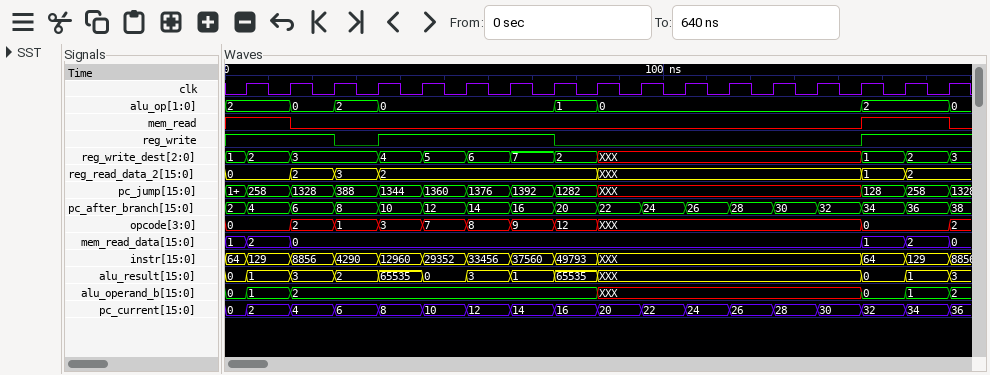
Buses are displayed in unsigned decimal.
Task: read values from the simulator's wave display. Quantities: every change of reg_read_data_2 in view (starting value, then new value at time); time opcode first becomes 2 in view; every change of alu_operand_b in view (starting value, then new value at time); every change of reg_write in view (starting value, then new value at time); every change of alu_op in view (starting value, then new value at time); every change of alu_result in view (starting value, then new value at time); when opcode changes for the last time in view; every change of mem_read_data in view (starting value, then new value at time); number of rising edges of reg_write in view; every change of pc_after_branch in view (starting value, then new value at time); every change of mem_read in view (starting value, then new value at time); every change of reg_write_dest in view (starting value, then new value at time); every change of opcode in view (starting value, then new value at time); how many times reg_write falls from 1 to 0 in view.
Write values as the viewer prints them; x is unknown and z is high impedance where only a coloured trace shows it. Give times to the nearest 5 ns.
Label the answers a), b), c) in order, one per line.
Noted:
a) 0, 2 at 15 ns, 3 at 25 ns, 2 at 35 ns, XXX at 85 ns, 1 at 145 ns, 2 at 155 ns
b) 15 ns
c) 0, 1 at 5 ns, 2 at 15 ns, XXX at 85 ns, 0 at 145 ns, 1 at 155 ns, 2 at 165 ns
d) 1, 0 at 25 ns, 1 at 35 ns, 0 at 75 ns, 1 at 145 ns
e) 2, 0 at 15 ns, 2 at 25 ns, 0 at 35 ns, 1 at 75 ns, 0 at 85 ns, 2 at 145 ns, 0 at 165 ns
f) 0, 1 at 5 ns, 3 at 15 ns, 2 at 25 ns, 65535 at 35 ns, 0 at 45 ns, 3 at 55 ns, 1 at 65 ns, 65535 at 75 ns, XXX at 85 ns, 0 at 145 ns, 1 at 155 ns, 3 at 165 ns
g) 165 ns
h) 1, 2 at 5 ns, 0 at 15 ns, 1 at 145 ns, 2 at 155 ns, 0 at 165 ns
i) 2
j) 2, 4 at 5 ns, 6 at 15 ns, 8 at 25 ns, 10 at 35 ns, 12 at 45 ns, 14 at 55 ns, 16 at 65 ns, 20 at 75 ns, 22 at 85 ns, 24 at 95 ns, 26 at 105 ns, 28 at 115 ns, 30 at 125 ns, 32 at 135 ns, 34 at 145 ns, 36 at 155 ns, 38 at 165 ns
k) 1, 0 at 15 ns, 1 at 145 ns, 0 at 165 ns
l) 1, 2 at 5 ns, 3 at 15 ns, 4 at 35 ns, 5 at 45 ns, 6 at 55 ns, 7 at 65 ns, 2 at 75 ns, XXX at 85 ns, 1 at 145 ns, 2 at 155 ns, 3 at 165 ns
m) 0, 2 at 15 ns, 1 at 25 ns, 3 at 35 ns, 7 at 45 ns, 8 at 55 ns, 9 at 65 ns, 12 at 75 ns, XXX at 85 ns, 0 at 145 ns, 2 at 165 ns
n) 2
